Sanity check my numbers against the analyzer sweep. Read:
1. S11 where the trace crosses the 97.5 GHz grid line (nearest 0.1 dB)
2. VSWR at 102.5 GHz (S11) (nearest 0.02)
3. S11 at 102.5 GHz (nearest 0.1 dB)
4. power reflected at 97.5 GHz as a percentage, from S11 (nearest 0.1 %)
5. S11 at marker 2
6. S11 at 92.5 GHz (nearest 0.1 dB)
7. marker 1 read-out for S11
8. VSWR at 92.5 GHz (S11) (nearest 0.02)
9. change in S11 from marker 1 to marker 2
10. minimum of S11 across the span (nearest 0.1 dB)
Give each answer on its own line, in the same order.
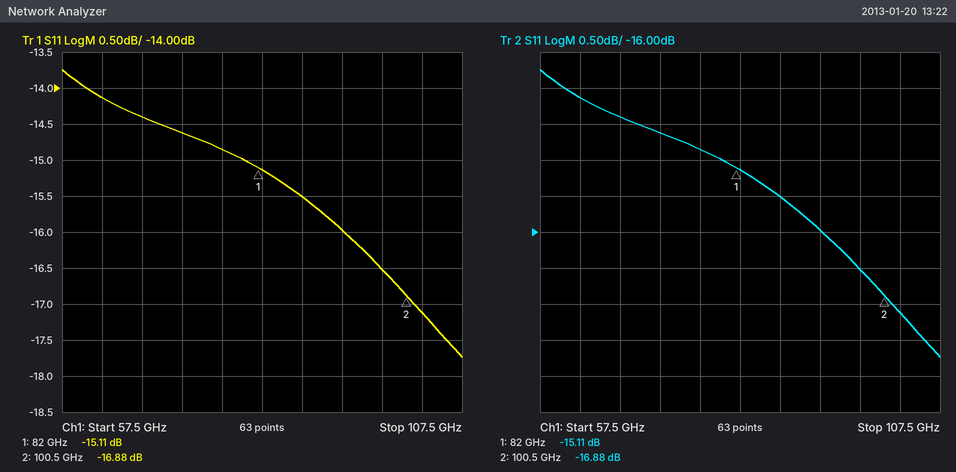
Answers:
-16.5 dB
1.32
-17.1 dB
2.2 %
-16.88 dB
-16.0 dB
-15.11 dB
1.38
-1.77 dB
-17.7 dB
